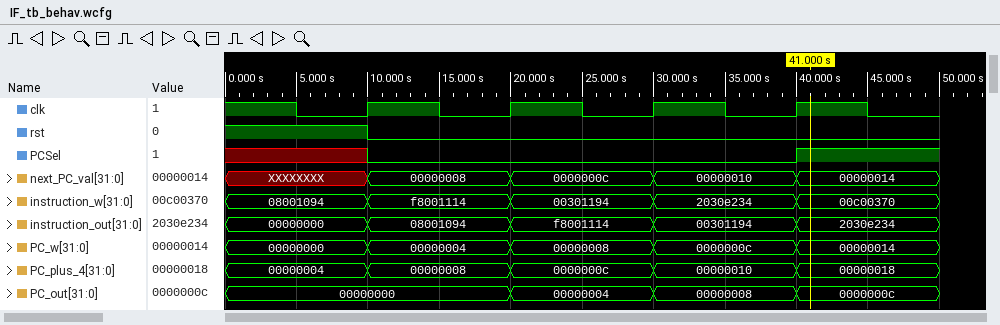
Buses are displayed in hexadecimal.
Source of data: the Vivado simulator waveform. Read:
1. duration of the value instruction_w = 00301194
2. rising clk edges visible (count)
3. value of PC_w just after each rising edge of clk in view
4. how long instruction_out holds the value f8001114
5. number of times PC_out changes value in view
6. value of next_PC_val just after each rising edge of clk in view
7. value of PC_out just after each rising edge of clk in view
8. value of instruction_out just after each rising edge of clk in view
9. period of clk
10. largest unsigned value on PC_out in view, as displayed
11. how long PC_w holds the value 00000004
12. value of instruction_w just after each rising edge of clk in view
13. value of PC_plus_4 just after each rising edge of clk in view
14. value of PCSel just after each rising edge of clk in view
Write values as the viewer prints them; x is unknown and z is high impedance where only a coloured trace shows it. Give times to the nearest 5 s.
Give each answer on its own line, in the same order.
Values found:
10 s
4
00000004, 00000008, 0000000c, 00000014
10 s
3
00000008, 0000000c, 00000010, 00000014
00000000, 00000004, 00000008, 0000000c
08001094, f8001114, 00301194, 2030e234
10 s
0000000c
10 s
f8001114, 00301194, 2030e234, 00c00370
00000008, 0000000c, 00000010, 00000018
0 0 0 1
